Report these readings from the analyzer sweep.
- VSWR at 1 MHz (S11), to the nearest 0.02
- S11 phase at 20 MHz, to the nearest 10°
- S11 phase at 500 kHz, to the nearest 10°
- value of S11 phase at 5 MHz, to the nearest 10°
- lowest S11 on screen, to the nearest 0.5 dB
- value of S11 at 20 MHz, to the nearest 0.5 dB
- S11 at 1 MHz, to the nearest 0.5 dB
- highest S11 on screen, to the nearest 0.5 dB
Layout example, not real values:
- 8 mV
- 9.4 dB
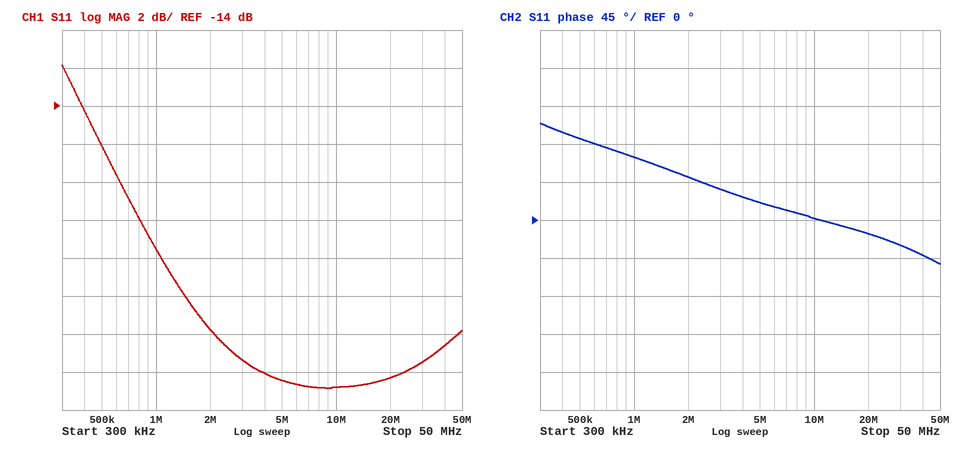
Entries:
- 1.18
- -20°
- 100°
- 20°
- -29.0 dB
- -28.5 dB
- -21.5 dB
- -12.0 dB
